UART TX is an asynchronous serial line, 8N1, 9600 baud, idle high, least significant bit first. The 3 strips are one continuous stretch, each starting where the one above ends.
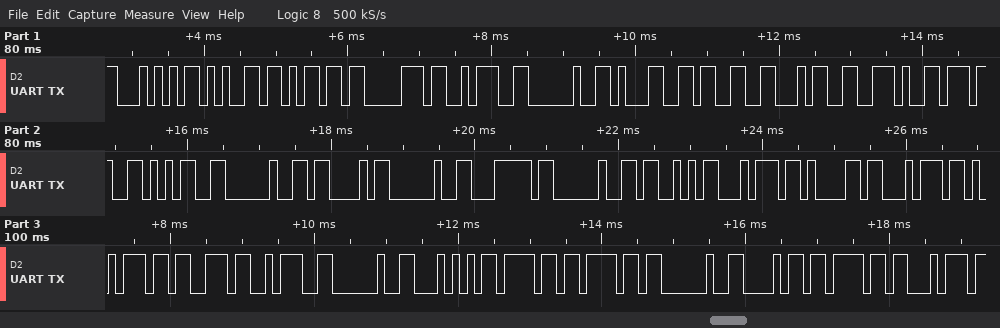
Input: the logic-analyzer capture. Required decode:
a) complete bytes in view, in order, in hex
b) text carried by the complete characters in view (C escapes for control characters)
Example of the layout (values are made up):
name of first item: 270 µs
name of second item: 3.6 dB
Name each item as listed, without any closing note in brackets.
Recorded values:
complete bytes in view, in order, in hex: 0x54 0x65 0x6D 0x70 0x3A 0x20 0x31 0x33 0x34 0x2E 0x37 0x35 0x20 0x43 0x20 0x7C 0x20 0x53 0x74 0x61 0x74 0x75 0x73 0x3A 0x20 0x54 0x6F 0x6F 0x20 0x68 0x6F 0x74
text carried by the complete characters in view: "Temp: 134.75 C | Status: Too hot"
